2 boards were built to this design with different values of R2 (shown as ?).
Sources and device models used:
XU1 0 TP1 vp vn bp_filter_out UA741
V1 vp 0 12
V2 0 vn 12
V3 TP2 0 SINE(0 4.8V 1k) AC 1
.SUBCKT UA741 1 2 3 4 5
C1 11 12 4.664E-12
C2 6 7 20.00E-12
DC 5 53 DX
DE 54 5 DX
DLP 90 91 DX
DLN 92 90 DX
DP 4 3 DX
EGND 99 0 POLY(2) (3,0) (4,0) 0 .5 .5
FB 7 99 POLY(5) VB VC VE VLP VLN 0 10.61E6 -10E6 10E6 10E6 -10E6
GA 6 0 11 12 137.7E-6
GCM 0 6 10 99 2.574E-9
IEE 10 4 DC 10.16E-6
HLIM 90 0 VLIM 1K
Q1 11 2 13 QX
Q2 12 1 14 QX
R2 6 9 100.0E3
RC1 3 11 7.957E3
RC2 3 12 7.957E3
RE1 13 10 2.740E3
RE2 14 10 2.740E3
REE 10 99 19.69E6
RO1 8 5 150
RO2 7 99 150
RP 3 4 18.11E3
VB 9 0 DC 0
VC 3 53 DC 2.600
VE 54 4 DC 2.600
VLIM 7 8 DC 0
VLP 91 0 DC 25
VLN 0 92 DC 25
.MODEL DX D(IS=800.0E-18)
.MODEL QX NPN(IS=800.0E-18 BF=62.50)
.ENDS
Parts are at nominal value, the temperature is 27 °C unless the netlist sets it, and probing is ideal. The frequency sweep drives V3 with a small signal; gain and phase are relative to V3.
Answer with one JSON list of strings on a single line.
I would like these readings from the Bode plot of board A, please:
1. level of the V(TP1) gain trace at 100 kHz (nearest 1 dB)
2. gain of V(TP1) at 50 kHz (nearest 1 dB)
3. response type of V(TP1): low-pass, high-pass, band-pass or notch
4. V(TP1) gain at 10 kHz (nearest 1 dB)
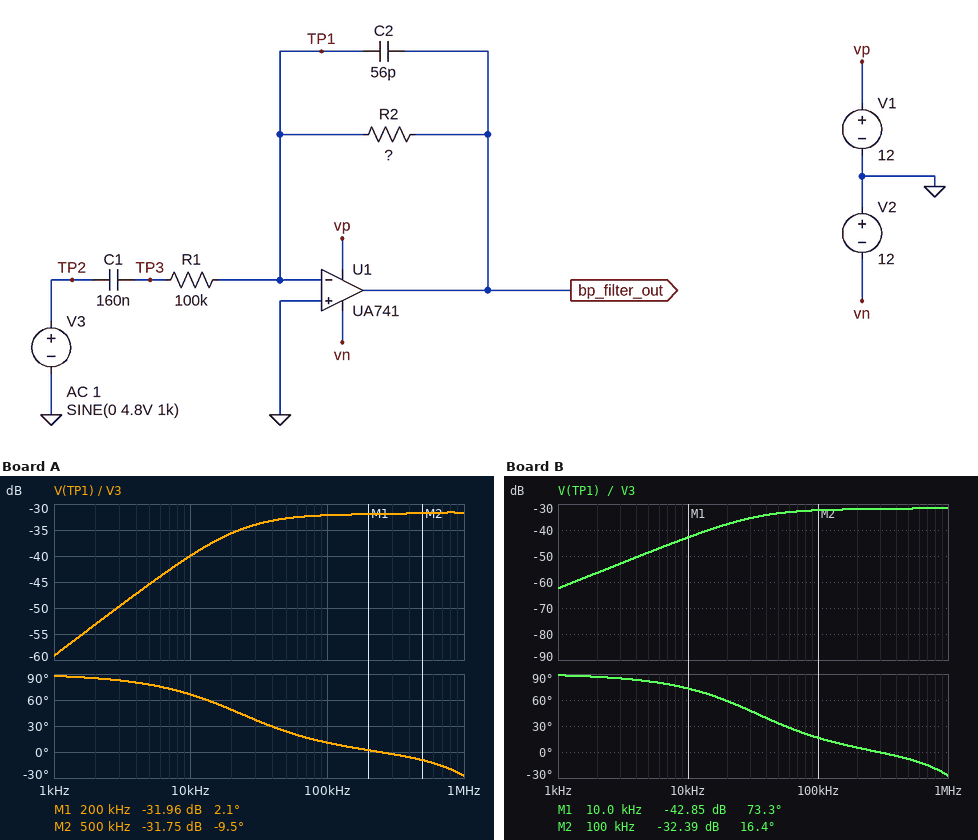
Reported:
["-32 dB", "-33 dB", "high-pass", "-40 dB"]
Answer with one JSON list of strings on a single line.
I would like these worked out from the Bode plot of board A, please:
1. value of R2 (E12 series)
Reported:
["120 kΩ"]
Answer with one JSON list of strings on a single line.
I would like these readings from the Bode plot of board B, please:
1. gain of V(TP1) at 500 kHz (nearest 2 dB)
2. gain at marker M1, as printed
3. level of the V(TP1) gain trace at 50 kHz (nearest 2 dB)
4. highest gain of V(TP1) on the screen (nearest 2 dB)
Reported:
["-32 dB", "-42.85 dB", "-34 dB", "-32 dB"]
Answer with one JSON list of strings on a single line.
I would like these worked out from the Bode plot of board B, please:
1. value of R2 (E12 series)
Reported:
["82 kΩ"]
